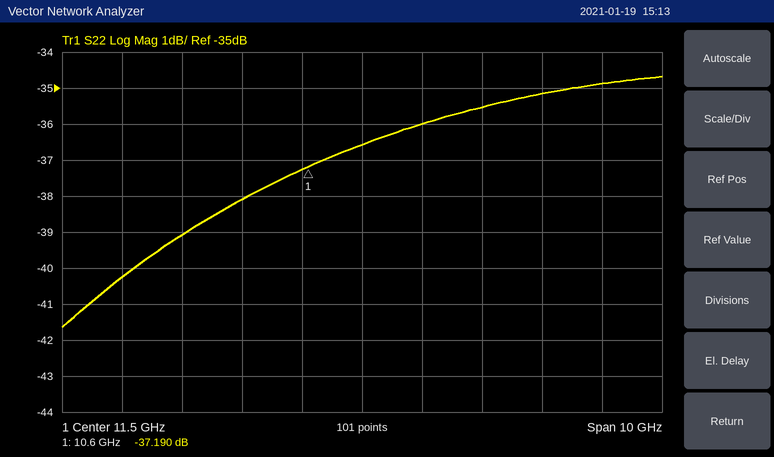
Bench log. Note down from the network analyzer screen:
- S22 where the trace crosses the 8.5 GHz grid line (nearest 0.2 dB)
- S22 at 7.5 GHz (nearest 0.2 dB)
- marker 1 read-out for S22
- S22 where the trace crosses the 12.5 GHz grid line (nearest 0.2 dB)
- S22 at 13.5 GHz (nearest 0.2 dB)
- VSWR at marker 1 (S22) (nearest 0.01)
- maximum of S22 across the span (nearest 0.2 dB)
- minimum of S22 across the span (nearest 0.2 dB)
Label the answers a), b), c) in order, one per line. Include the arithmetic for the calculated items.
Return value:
a) -39.0 dB
b) -40.2 dB
c) -37.190 dB
d) -36.0 dB
e) -35.6 dB
f) (1 + 0.0138)/(1 − 0.0138) ≈ 1.03
g) -34.6 dB
h) -41.6 dB
